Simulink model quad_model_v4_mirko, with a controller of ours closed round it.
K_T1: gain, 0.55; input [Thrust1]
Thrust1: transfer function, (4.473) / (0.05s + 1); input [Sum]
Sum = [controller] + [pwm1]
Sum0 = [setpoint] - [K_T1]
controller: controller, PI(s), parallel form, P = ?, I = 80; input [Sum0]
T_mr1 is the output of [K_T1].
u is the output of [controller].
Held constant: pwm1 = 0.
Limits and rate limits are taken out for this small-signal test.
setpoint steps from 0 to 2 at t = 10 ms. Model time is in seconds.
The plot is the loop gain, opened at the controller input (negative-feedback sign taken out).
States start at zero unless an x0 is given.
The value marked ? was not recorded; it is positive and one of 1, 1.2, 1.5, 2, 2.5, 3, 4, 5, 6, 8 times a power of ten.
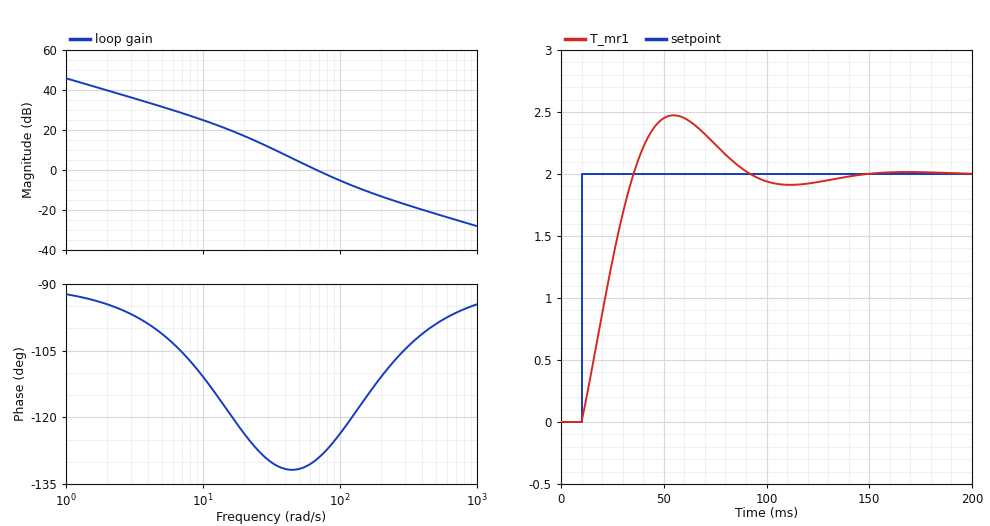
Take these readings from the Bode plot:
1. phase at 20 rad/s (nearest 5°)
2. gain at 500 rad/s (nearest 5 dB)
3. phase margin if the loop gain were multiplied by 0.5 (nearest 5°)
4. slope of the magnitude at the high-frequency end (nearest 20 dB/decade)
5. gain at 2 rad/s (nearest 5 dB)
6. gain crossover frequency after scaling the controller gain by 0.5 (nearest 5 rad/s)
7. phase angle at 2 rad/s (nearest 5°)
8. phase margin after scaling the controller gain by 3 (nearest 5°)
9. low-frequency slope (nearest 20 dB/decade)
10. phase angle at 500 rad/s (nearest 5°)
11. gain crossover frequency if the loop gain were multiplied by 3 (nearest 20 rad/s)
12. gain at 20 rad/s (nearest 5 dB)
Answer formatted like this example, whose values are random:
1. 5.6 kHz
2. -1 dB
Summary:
1. -125°
2. -20 dB
3. 50°
4. -20 dB/decade
5. 40 dB
6. 45 rad/s
7. -95°
8. 65°
9. -20 dB/decade
10. -100°
11. 140 rad/s
12. 15 dB
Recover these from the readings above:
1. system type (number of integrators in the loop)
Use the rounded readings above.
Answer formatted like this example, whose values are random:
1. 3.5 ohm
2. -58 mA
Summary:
1. 1
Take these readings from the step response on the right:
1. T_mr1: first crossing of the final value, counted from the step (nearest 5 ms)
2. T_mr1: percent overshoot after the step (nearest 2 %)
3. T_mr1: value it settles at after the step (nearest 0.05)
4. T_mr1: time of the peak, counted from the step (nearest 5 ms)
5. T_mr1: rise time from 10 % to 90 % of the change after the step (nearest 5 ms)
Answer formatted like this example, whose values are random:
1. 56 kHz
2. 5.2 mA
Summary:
1. 25 ms
2. 24 %
3. 2.00
4. 45 ms
5. 20 ms
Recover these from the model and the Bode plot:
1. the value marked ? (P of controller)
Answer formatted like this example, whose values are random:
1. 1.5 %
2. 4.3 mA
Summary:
1. 0.8
